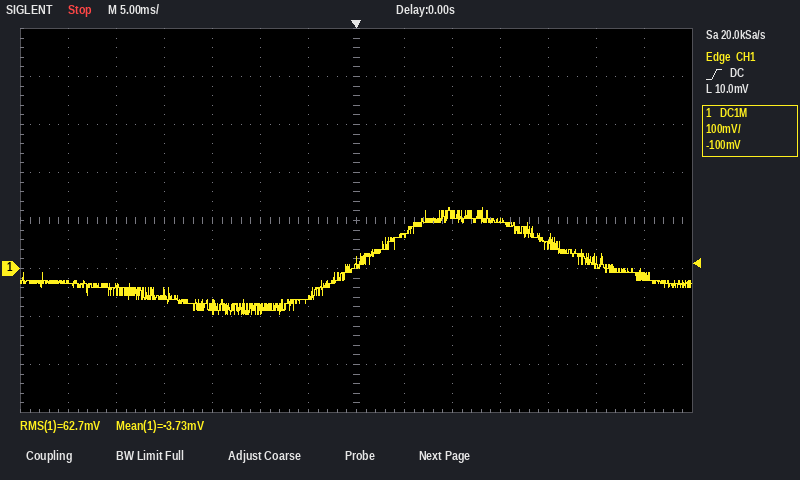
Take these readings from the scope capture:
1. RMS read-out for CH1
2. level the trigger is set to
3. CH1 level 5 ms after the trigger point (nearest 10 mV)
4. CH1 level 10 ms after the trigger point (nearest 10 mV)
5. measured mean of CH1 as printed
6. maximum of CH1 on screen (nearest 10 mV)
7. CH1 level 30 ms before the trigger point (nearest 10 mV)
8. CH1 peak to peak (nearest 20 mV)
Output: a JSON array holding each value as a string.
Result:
["62.7 mV", "10.0 mV", "70 mV", "110 mV", "-3.73 mV", "130 mV", "-30 mV", "220 mV"]
